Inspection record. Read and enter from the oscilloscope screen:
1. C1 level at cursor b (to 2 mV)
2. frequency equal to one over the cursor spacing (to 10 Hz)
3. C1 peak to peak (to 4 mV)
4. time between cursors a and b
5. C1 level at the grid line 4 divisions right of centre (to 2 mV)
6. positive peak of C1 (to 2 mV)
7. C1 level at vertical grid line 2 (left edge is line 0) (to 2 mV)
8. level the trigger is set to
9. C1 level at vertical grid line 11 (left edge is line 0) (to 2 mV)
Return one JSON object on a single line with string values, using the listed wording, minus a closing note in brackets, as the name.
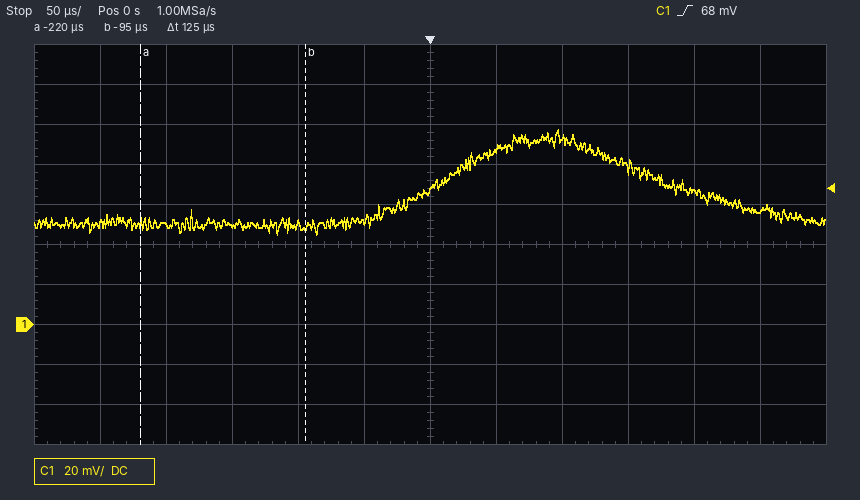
{"C1 level at cursor b": "50 mV", "frequency equal to one over the cursor spacing": "8.00 kHz", "C1 peak to peak": "52 mV", "time between cursors a and b": "125 µs", "C1 level at the grid line 4 divisions right of centre": "66 mV", "positive peak of C1": "98 mV", "C1 level at vertical grid line 2 (left edge is line 0)": "50 mV", "level the trigger is set to": "68 mV", "C1 level at vertical grid line 11 (left edge is line 0)": "58 mV"}
